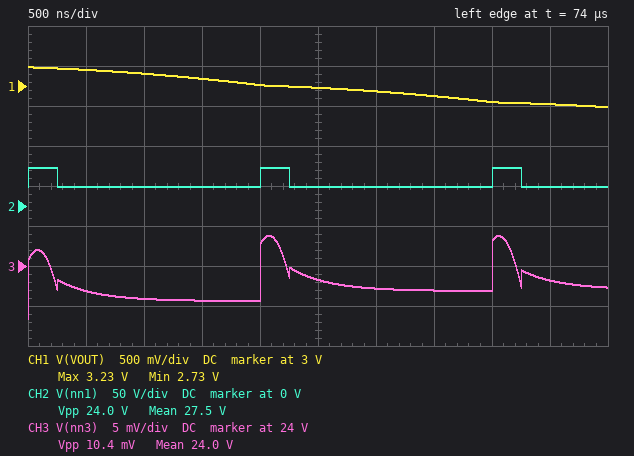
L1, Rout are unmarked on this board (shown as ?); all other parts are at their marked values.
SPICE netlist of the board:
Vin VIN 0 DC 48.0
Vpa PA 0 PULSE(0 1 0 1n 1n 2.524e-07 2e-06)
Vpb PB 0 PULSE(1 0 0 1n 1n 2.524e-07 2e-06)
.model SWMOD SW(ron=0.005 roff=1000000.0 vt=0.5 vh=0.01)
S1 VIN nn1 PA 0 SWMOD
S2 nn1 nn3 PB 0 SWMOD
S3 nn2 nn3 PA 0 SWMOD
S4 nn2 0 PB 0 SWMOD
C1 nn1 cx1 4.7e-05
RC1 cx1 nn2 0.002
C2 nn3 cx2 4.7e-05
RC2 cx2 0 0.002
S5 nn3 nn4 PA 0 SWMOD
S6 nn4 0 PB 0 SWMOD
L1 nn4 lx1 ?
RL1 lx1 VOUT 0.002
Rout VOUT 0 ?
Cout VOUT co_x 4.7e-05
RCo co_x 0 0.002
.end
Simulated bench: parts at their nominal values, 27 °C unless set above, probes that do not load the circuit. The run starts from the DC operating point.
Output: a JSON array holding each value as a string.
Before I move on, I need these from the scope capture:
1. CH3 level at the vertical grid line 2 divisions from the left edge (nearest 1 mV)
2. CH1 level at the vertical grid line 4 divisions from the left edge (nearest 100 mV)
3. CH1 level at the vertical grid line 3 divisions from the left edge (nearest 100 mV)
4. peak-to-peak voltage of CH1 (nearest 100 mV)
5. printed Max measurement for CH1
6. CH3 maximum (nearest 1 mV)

["24.001 V", "3.0 V", "3.1 V", "500 mV", "3.23 V", "24.009 V"]
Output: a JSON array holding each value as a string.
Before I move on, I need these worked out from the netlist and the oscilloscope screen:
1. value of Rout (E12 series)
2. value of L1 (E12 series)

["0.82 Ω", "1 µH"]
